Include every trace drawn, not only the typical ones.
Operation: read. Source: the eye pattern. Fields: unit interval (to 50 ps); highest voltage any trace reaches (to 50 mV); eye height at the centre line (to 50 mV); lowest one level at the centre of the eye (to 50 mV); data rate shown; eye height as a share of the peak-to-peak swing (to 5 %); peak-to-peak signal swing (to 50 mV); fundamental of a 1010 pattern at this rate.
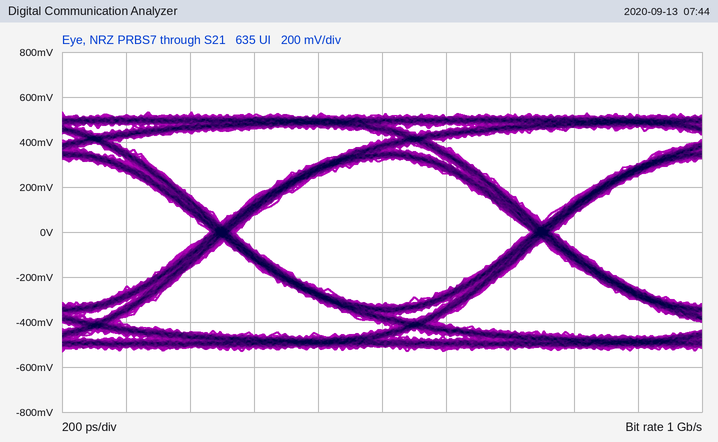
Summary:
1.00 ns
550 mV
650 mV
300 mV
1 Gb/s
60 %
1.05 V
500 MHz
